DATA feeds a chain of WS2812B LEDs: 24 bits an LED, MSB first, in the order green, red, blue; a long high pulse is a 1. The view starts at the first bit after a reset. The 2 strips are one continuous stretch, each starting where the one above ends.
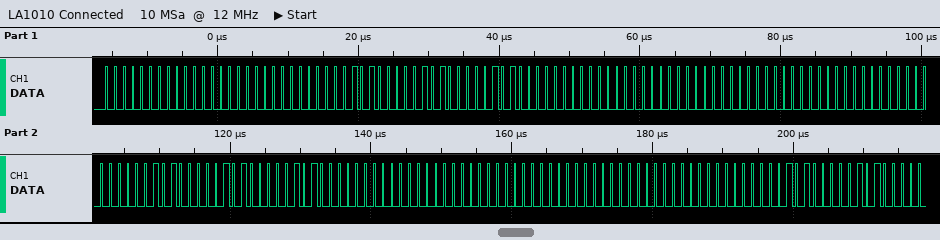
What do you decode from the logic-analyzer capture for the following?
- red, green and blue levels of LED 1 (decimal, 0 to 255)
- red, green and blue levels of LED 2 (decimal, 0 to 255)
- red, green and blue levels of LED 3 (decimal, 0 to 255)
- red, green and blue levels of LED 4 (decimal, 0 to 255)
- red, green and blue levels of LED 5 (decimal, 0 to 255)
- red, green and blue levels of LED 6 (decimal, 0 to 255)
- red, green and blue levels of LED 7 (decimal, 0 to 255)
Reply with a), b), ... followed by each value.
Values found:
a) 0, 0, 0
b) 10, 10, 10
c) 0, 0, 0
d) 0, 0, 0
e) 10, 10, 10
f) 0, 0, 0
g) 0, 0, 0
